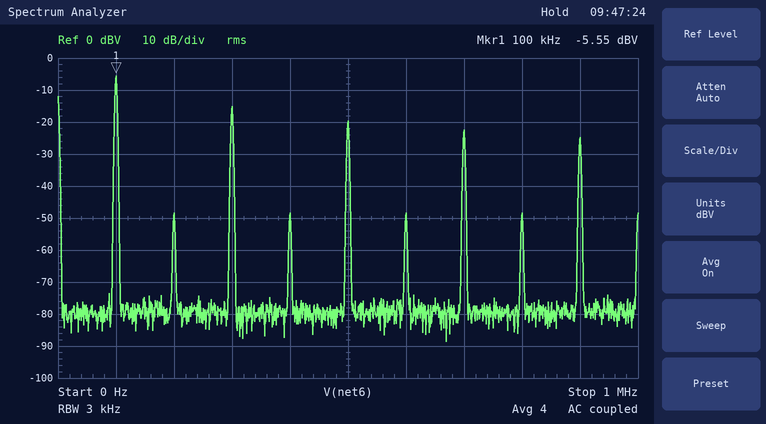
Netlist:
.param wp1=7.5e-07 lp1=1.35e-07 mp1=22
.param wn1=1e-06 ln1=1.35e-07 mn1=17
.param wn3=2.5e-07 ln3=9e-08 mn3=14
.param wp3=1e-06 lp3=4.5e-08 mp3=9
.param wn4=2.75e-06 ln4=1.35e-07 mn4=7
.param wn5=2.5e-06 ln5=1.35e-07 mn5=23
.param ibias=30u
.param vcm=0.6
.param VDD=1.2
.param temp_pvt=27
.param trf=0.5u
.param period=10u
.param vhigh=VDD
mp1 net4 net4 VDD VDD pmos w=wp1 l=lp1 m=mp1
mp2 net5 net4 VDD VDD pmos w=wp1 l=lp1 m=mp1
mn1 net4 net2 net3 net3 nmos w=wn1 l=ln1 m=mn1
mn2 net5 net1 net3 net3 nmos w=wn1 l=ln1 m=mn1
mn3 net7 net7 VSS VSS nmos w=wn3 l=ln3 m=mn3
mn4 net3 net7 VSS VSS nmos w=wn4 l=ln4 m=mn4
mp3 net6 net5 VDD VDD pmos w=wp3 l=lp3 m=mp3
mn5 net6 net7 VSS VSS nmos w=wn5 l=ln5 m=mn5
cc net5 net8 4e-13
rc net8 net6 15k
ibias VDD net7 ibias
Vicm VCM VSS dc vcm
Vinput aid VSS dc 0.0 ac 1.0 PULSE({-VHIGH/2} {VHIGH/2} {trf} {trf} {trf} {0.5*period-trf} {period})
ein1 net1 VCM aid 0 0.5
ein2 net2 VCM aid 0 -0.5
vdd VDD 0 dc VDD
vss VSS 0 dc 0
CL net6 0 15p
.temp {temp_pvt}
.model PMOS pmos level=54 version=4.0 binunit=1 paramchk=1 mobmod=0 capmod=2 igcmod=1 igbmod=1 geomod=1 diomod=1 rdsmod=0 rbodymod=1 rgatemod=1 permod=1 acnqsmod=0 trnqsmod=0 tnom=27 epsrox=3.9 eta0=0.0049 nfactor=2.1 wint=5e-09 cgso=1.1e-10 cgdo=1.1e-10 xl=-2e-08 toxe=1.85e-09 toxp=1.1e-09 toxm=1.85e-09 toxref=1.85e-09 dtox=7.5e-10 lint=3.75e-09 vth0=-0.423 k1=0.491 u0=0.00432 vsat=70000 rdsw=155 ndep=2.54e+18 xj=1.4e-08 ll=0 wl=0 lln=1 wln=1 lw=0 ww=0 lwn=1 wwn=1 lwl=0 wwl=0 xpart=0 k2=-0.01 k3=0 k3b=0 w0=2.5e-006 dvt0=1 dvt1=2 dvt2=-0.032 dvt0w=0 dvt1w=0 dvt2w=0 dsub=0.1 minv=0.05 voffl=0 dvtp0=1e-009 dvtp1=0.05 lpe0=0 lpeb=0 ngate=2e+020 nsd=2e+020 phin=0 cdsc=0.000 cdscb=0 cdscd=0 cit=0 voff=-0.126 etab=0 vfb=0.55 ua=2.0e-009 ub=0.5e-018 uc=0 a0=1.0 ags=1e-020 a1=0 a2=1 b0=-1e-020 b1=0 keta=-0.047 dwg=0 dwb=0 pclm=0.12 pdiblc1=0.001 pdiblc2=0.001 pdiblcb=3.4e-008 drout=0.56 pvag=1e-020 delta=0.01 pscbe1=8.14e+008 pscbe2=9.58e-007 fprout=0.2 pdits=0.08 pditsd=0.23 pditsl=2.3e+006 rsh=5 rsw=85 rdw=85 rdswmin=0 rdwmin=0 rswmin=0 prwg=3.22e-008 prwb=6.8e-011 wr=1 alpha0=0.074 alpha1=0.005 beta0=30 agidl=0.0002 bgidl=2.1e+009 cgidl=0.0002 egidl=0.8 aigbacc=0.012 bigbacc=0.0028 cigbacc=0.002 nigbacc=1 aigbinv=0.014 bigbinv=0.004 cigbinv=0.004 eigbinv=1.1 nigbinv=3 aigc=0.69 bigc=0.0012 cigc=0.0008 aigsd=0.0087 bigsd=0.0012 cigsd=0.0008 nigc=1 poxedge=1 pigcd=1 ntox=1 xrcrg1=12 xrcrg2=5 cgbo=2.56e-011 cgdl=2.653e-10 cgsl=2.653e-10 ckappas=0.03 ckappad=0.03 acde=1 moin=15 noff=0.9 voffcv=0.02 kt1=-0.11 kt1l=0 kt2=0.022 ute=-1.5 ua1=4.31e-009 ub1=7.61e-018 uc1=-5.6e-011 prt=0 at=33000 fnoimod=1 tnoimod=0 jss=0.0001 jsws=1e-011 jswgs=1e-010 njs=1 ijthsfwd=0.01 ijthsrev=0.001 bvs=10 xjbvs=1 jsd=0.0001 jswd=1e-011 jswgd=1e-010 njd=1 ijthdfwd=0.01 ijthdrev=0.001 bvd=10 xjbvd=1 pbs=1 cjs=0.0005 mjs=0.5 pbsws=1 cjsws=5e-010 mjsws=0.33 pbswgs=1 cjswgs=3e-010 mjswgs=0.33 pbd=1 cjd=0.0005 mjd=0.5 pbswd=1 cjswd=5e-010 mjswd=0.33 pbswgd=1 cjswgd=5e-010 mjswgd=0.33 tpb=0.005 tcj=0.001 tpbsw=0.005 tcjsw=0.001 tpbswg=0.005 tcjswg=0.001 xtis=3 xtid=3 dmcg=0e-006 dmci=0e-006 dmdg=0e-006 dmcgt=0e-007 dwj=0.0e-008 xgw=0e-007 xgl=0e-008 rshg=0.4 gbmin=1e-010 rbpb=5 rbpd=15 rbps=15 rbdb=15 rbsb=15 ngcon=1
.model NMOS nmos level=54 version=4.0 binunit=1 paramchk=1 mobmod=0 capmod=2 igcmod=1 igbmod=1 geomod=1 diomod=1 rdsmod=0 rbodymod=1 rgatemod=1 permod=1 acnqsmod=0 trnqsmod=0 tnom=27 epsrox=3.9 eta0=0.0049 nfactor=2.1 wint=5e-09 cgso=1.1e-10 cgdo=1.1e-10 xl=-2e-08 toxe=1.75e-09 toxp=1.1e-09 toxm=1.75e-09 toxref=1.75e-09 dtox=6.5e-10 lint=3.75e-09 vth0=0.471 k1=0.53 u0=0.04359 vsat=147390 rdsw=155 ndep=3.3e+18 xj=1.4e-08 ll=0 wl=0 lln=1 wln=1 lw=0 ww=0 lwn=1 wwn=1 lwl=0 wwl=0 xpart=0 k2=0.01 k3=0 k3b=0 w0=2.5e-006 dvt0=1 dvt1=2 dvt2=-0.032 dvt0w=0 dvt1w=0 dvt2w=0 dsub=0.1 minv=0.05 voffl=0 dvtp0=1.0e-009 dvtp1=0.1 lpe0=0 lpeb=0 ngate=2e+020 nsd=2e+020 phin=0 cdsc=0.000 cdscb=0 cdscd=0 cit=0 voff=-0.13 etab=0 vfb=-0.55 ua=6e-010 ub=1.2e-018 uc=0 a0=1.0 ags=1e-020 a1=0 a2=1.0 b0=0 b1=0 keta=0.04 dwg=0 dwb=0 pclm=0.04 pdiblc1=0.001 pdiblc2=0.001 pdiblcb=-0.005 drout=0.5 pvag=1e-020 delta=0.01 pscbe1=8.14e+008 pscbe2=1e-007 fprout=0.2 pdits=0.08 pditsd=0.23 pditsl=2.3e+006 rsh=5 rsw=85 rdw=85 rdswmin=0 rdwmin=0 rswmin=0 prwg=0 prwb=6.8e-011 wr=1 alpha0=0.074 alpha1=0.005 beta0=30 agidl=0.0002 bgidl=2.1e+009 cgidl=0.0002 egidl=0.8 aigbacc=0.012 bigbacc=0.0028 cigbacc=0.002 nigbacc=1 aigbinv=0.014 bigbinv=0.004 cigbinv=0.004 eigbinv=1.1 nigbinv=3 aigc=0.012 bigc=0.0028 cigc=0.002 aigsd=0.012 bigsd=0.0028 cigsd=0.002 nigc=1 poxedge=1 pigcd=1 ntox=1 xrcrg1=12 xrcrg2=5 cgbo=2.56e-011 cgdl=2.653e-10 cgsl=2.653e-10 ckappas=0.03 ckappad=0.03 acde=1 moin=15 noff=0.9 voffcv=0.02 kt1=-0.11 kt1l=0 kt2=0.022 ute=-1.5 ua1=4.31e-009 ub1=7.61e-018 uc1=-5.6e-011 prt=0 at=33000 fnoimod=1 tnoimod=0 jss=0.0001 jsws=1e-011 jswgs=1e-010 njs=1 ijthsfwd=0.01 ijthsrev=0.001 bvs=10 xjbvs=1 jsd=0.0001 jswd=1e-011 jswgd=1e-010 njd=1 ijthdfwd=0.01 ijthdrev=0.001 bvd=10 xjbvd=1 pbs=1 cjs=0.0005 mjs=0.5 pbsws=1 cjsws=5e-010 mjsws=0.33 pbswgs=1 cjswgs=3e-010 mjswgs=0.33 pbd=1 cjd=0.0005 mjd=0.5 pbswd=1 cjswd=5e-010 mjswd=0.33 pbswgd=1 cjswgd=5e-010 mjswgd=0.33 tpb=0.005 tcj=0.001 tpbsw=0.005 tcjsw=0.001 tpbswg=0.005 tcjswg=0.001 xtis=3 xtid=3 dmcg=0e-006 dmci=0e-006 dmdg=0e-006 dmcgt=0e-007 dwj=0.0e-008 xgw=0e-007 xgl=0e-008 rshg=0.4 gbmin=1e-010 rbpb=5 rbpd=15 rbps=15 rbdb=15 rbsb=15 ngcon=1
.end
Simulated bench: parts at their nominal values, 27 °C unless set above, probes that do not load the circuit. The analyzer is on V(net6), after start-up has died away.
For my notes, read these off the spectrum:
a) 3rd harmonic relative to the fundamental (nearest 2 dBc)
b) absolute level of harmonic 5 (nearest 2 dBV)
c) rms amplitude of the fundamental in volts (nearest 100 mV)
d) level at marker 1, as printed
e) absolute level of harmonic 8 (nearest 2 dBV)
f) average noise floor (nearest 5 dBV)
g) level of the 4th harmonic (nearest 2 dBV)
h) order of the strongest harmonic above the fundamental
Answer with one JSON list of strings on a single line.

["-10 dBc", "-20 dBV", "500 mV", "-5.55 dBV", "-48 dBV", "-80 dBV", "-48 dBV", "3"]
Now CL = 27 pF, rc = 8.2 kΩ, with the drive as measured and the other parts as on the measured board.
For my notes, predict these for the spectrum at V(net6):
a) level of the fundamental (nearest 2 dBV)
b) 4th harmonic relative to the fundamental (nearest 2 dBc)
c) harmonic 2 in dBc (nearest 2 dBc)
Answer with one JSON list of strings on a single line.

["-6 dBV", "-38 dBc", "-38 dBc"]
